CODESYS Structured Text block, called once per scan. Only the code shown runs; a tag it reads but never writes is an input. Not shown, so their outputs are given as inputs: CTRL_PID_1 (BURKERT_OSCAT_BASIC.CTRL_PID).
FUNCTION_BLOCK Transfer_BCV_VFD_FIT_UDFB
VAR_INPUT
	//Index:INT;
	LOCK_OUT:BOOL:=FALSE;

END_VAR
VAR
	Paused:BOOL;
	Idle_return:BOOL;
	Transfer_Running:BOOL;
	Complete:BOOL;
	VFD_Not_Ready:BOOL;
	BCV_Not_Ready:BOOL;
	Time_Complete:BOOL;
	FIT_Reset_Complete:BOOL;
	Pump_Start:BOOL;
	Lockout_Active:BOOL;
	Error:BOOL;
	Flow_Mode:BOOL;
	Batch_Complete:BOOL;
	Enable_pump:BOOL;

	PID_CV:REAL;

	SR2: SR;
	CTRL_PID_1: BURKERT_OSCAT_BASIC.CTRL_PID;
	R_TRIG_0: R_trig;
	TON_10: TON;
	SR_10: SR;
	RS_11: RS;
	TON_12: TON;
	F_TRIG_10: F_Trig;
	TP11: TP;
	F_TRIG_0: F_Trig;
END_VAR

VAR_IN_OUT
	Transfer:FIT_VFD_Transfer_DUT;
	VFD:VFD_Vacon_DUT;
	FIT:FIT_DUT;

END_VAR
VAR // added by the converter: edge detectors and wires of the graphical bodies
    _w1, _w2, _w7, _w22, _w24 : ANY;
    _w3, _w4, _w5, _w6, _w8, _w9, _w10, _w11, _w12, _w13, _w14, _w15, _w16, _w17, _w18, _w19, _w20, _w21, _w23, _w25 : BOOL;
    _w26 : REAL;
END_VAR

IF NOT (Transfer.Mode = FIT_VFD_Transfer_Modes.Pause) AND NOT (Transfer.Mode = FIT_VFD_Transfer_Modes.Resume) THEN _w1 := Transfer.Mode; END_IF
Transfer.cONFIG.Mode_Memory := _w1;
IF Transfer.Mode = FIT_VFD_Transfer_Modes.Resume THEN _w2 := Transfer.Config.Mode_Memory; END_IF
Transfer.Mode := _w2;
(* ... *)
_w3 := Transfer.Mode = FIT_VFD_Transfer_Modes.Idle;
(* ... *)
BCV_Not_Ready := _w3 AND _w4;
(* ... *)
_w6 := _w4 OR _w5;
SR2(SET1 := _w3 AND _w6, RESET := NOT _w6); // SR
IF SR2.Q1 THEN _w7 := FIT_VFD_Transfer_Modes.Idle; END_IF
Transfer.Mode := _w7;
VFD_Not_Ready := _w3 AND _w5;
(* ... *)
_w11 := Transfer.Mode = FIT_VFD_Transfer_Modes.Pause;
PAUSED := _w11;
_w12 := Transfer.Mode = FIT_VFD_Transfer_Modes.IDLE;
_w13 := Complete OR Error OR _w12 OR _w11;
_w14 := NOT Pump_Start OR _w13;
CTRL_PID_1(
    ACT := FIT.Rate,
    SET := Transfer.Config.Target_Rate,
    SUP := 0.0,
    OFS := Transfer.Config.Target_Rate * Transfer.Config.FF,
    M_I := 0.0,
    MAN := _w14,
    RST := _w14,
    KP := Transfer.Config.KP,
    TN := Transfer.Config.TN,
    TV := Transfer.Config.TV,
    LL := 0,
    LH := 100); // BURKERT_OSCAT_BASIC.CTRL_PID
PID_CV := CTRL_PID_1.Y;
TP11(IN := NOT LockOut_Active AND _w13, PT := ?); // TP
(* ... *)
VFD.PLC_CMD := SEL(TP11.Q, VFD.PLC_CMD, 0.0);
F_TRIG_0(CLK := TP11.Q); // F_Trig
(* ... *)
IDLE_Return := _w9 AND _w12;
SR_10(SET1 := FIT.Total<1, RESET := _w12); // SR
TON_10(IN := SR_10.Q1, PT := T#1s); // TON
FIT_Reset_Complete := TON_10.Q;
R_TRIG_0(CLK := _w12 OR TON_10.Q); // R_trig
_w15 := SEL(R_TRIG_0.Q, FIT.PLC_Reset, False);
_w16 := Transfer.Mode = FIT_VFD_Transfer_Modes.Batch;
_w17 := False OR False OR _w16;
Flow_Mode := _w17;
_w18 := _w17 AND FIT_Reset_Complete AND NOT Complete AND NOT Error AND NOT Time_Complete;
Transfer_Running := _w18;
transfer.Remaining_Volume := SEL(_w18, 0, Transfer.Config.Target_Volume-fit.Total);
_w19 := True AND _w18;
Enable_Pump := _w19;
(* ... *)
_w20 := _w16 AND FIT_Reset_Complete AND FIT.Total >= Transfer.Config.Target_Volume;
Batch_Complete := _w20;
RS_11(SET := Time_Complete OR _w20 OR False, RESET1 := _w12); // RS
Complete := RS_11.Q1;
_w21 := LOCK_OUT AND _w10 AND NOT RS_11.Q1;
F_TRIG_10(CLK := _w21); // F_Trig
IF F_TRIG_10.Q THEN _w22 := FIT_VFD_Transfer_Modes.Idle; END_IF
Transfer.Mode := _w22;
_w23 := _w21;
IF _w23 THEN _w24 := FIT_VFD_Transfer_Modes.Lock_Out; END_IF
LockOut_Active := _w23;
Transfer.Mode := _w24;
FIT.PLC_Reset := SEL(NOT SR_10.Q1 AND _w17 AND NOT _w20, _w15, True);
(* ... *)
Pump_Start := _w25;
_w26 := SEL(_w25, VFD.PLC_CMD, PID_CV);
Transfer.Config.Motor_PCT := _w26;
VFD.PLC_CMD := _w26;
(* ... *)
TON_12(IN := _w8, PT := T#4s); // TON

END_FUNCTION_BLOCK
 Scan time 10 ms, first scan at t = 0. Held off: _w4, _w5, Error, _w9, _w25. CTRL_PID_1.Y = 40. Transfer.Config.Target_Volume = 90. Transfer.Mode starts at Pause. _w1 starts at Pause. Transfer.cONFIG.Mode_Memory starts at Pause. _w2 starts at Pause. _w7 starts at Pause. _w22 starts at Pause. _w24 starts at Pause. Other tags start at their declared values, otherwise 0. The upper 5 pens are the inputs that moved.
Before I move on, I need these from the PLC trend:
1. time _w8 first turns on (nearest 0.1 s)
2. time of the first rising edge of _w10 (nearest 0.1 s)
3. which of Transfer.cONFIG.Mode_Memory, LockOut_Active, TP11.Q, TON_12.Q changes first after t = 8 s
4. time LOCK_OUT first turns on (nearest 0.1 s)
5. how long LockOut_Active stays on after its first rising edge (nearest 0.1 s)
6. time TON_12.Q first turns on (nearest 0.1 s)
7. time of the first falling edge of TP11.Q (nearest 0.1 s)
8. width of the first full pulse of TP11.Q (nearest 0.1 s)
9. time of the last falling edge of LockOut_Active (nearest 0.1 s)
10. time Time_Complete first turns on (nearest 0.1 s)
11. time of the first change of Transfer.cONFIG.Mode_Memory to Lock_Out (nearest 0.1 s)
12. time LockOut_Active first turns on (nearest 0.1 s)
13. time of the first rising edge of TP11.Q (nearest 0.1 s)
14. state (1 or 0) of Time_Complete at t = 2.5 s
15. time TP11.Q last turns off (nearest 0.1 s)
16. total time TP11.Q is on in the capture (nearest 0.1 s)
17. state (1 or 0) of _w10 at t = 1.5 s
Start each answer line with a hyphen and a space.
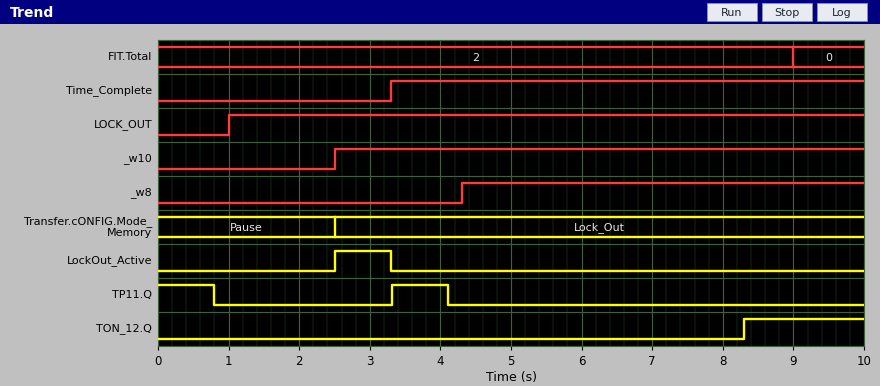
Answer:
- 4.3 s
- 2.5 s
- TON_12.Q
- 1.0 s
- 0.8 s
- 8.3 s
- 0.8 s
- 0.8 s
- 3.3 s
- 3.3 s
- 2.5 s
- 2.5 s
- 3.3 s
- 0
- 4.1 s
- 1.6 s
- 0
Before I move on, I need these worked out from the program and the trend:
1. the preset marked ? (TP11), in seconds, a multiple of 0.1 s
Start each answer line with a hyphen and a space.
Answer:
- 0.8 s
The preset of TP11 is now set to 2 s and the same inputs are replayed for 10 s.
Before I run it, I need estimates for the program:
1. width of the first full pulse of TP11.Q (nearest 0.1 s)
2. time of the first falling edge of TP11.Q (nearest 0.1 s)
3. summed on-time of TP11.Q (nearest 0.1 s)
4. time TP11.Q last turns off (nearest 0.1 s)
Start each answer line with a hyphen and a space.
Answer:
- 2.0 s
- 2.0 s
- 4.0 s
- 5.3 s
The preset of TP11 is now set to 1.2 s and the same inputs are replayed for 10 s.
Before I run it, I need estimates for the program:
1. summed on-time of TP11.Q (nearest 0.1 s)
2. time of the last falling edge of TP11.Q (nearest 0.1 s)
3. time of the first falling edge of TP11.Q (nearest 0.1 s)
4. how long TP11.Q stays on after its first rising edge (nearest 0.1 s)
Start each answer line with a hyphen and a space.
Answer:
- 2.4 s
- 4.5 s
- 1.2 s
- 1.2 s
